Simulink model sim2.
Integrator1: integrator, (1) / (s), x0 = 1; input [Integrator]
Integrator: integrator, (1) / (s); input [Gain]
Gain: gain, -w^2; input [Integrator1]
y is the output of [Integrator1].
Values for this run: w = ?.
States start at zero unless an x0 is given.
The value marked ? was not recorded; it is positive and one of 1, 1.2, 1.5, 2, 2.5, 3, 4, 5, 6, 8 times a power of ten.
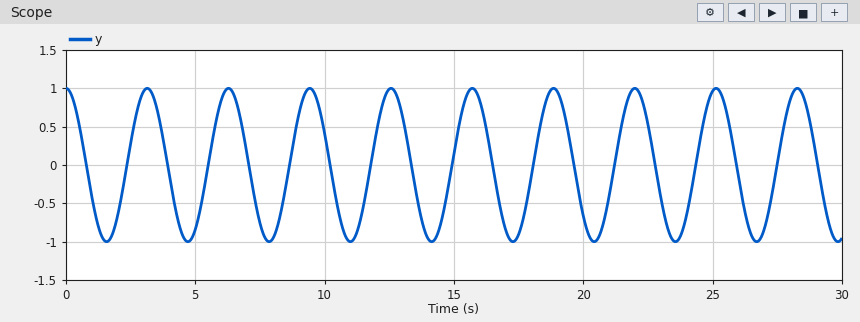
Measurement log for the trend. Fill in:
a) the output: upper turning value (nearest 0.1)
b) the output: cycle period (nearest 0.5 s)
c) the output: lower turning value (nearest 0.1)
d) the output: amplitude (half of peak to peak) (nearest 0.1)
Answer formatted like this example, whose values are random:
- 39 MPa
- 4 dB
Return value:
- 1.0
- 3.0 s
- -1.0
- 1.0
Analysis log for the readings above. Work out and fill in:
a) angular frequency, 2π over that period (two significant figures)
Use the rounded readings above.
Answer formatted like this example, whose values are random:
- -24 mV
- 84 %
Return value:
- 2.1 rad/s
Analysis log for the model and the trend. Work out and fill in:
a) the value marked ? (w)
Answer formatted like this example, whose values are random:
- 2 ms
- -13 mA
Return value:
- 2
